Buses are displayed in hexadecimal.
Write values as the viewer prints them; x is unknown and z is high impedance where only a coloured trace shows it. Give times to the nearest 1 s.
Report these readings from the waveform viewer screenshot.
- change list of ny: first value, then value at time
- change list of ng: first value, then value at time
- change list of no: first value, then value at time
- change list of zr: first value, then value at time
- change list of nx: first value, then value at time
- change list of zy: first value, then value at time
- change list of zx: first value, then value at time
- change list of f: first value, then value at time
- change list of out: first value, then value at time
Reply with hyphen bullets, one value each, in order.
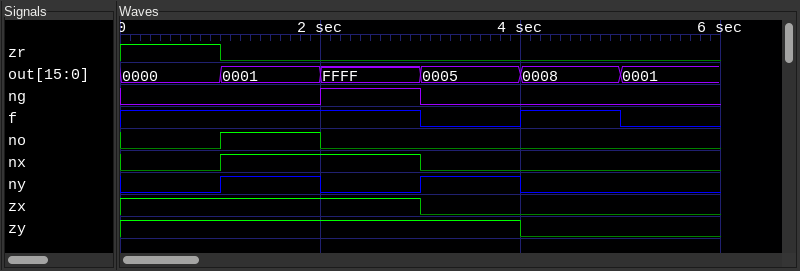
- 0, 1 at 1 s, 0 at 2 s, 1 at 3 s, 0 at 4 s
- 0, 1 at 2 s, 0 at 3 s
- 0, 1 at 1 s, 0 at 2 s
- 1, 0 at 1 s
- 0, 1 at 1 s, 0 at 3 s
- 1, 0 at 4 s
- 1, 0 at 3 s
- 1, 0 at 3 s, 1 at 4 s, 0 at 5 s
- 0000, 0001 at 1 s, FFFF at 2 s, 0005 at 3 s, 0008 at 4 s, 0001 at 5 s
